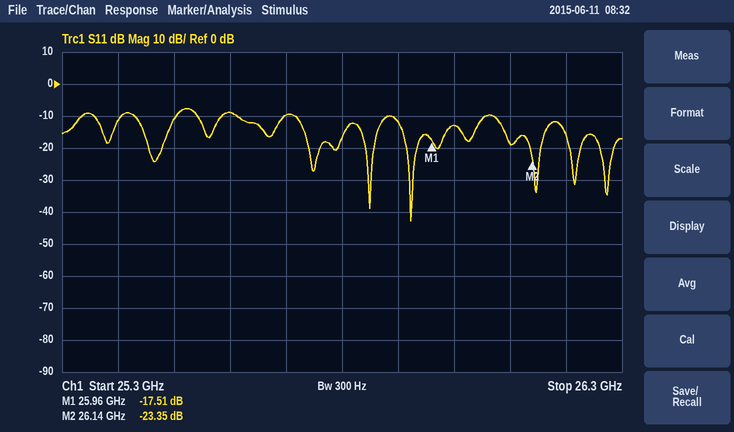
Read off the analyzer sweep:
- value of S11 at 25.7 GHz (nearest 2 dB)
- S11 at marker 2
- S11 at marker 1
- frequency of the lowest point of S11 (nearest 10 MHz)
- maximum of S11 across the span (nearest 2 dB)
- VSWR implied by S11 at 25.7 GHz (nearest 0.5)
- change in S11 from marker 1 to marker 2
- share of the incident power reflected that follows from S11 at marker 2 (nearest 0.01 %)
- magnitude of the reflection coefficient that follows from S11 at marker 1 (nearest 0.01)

-10 dB
-23.35 dB
-17.51 dB
25.92 GHz
-8 dB
2.0
-5.84 dB
0.46 %
0.13
